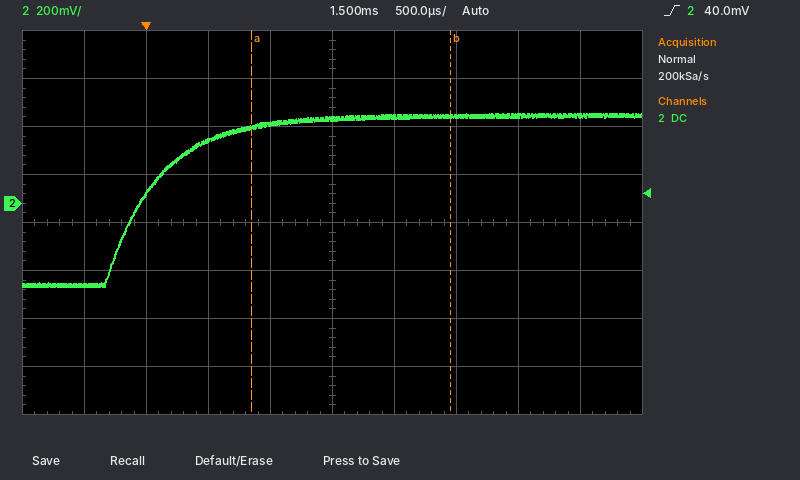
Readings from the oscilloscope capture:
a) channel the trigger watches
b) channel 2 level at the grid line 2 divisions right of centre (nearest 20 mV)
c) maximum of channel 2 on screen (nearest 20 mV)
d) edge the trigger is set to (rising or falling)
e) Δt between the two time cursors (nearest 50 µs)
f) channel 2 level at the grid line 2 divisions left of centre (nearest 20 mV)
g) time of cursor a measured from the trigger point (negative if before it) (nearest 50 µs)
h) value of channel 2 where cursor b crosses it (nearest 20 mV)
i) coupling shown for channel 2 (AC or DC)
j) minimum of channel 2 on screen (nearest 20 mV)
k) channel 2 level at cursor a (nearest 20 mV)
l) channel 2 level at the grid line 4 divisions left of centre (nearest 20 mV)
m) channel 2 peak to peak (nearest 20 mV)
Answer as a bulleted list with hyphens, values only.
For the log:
- channel 2
- 360 mV
- 380 mV
- rising
- 1.60 ms
- 260 mV
- +850 µs
- 360 mV
- DC
- -340 mV
- 320 mV
- -340 mV
- 720 mV
